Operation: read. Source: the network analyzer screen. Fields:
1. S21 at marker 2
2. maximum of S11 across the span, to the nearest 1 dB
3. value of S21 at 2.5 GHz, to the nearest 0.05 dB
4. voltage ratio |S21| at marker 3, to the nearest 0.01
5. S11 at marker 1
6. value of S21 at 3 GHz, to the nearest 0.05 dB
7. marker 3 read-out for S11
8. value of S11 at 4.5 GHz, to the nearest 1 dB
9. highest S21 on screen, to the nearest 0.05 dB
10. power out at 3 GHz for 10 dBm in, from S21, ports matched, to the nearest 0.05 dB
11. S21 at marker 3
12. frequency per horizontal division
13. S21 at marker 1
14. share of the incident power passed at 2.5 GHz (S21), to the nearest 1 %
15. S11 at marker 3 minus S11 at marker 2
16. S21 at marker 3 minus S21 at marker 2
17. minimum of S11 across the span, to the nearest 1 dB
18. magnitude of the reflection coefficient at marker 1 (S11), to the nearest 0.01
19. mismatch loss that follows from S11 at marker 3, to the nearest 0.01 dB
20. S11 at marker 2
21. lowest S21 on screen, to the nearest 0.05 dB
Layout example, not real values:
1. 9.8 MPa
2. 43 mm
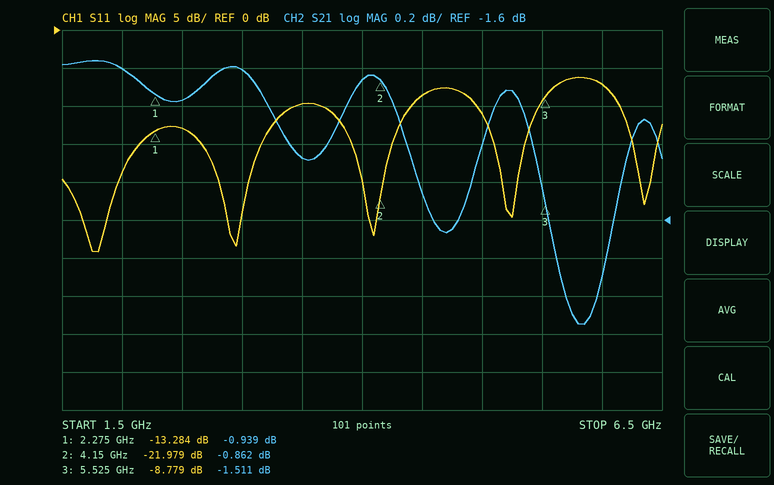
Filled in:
1. -0.862 dB
2. -6 dB
3. -0.95 dB
4. 0.84
5. -13.284 dB
6. -0.80 dB
7. -8.779 dB
8. -9 dB
9. -0.75 dB
10. 9.20 dBm
11. -1.511 dB
12. 500 MHz
13. -0.939 dB
14. 80 %
15. 13.200 dB
16. -0.649 dB
17. -29 dB
18. 0.22
19. 0.62 dB
20. -21.979 dB
21. -2.15 dB
